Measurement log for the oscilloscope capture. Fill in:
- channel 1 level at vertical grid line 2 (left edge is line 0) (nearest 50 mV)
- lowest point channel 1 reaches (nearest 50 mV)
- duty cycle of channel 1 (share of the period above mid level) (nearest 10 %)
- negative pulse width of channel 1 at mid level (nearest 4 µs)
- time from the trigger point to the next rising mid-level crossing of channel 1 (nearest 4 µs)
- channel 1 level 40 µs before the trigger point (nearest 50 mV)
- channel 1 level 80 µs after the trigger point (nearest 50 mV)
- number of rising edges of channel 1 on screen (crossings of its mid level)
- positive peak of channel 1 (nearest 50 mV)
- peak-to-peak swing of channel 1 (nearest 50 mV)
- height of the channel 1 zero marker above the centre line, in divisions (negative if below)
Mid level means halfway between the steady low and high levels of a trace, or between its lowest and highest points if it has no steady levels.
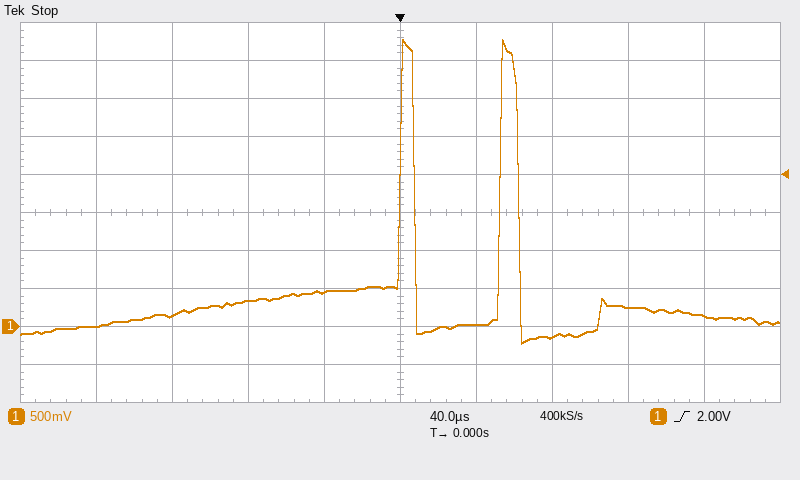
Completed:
150 mV
-200 mV
20 %
44 µs
52 µs
450 mV
-150 mV
2
3.80 V
4.00 V
-3.0 div
